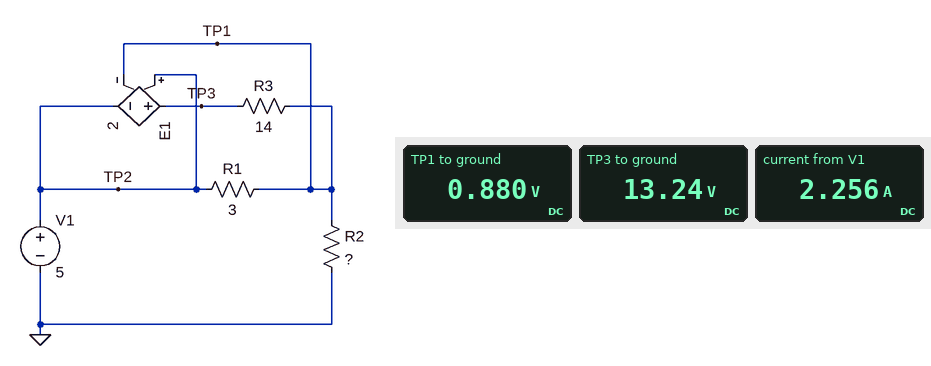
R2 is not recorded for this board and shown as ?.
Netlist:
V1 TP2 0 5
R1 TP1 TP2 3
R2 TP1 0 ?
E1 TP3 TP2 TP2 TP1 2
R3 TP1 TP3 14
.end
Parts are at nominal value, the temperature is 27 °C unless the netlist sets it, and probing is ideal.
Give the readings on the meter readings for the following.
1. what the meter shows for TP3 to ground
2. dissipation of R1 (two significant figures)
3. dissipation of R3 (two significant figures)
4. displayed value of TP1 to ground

13.24 V
5.7 W
11 W
0.880 V
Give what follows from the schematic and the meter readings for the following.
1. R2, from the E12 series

0.39 Ω
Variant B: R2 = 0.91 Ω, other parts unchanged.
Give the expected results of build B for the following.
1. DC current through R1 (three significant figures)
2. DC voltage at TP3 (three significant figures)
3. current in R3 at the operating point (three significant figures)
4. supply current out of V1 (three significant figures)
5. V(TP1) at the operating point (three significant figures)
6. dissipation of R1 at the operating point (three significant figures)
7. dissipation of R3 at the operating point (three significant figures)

1.11 A
11.7 V
715 mA
1.83 A
1.66 V
3.71 W
7.16 W
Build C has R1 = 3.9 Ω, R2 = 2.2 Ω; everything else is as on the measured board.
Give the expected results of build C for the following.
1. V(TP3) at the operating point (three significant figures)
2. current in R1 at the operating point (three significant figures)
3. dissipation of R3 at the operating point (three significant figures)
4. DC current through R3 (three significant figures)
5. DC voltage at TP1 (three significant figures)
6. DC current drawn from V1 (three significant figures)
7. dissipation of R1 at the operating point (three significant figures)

9.91 V
630 mA
3.88 W
526 mA
2.54 V
1.16 A
1.55 W
